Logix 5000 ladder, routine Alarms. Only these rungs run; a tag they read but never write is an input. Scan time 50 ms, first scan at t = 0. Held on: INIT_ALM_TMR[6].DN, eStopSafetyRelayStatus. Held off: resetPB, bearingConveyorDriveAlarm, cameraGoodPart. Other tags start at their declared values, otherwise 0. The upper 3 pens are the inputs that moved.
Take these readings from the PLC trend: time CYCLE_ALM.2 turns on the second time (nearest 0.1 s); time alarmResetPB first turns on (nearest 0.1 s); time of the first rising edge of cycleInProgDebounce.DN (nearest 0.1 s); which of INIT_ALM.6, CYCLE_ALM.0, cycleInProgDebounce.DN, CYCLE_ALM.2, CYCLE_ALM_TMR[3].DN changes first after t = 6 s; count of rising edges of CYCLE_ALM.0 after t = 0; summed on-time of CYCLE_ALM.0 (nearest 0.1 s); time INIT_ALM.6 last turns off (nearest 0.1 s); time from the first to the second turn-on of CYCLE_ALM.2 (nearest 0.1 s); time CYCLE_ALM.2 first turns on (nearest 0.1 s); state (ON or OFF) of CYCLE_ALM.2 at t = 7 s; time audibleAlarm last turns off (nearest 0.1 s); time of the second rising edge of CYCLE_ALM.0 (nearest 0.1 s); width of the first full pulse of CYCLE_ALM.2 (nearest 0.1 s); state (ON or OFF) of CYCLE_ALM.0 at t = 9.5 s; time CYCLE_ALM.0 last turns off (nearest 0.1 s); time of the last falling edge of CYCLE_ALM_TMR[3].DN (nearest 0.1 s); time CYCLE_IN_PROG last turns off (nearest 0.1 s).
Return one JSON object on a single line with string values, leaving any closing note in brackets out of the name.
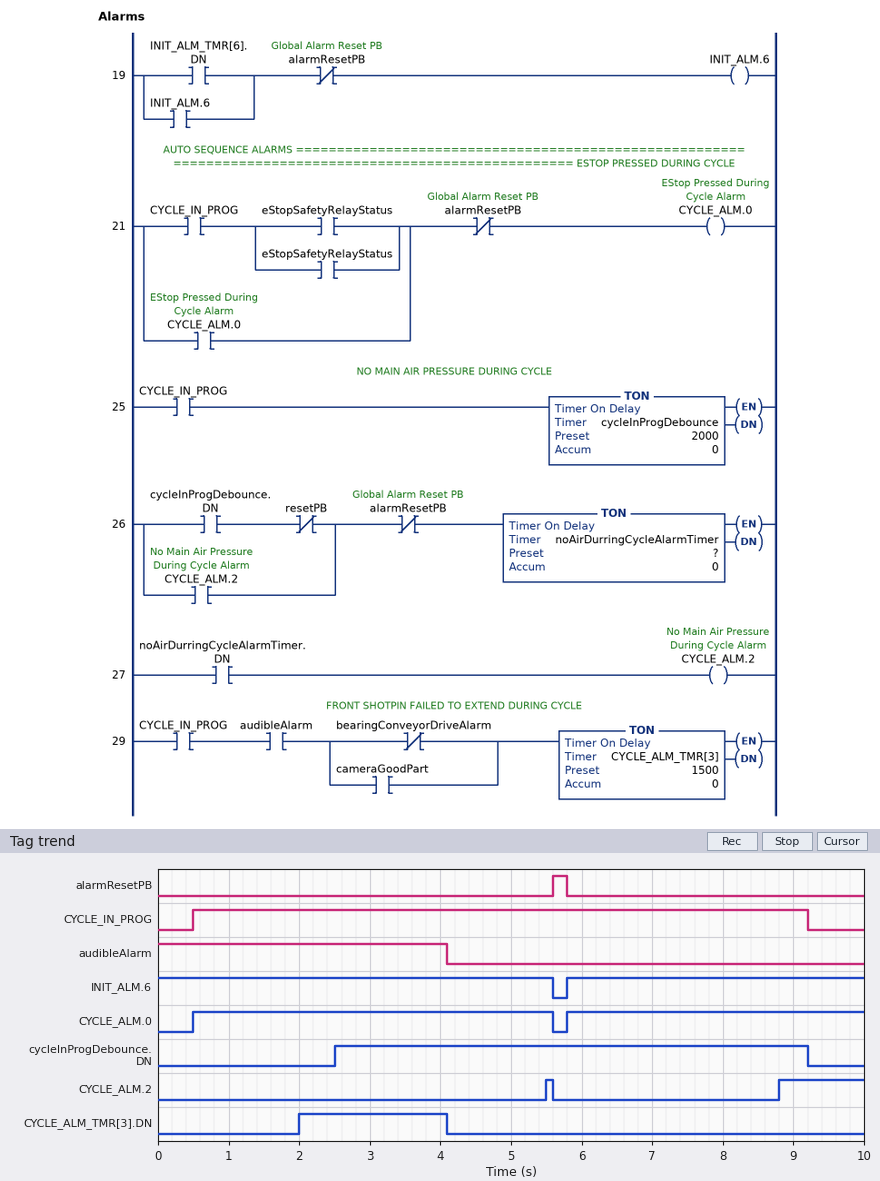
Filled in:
{"time CYCLE_ALM.2 turns on the second time": "8.8 s", "time alarmResetPB first turns on": "5.6 s", "time of the first rising edge of cycleInProgDebounce.DN": "2.5 s", "which of INIT_ALM.6, CYCLE_ALM.0, cycleInProgDebounce.DN, CYCLE_ALM.2, CYCLE_ALM_TMR[3].DN changes first after t = 6 s": "CYCLE_ALM.2", "count of rising edges of CYCLE_ALM.0 after t = 0": "2", "summed on-time of CYCLE_ALM.0": "9.3 s", "time INIT_ALM.6 last turns off": "5.6 s", "time from the first to the second turn-on of CYCLE_ALM.2": "3.3 s", "time CYCLE_ALM.2 first turns on": "5.5 s", "state (ON or OFF) of CYCLE_ALM.2 at t = 7 s": "OFF", "time audibleAlarm last turns off": "4.1 s", "time of the second rising edge of CYCLE_ALM.0": "5.8 s", "width of the first full pulse of CYCLE_ALM.2": "0.1 s", "state (ON or OFF) of CYCLE_ALM.0 at t = 9.5 s": "ON", "time CYCLE_ALM.0 last turns off": "5.6 s", "time of the last falling edge of CYCLE_ALM_TMR[3].DN": "4.1 s", "time CYCLE_IN_PROG last turns off": "9.2 s"}
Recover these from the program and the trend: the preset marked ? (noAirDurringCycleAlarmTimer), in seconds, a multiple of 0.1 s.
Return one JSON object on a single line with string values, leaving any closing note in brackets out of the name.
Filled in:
{"the preset marked ? (noAirDurringCycleAlarmTimer), in seconds, a multiple of 0.1 s": "3.0 s"}
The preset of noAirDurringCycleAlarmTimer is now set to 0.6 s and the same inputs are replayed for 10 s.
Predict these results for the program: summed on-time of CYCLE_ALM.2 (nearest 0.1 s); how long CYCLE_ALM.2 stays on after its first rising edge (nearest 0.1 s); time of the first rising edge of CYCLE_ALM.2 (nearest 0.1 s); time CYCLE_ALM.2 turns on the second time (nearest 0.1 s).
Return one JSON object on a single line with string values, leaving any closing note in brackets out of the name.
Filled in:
{"summed on-time of CYCLE_ALM.2": "6.1 s", "how long CYCLE_ALM.2 stays on after its first rising edge": "2.5 s", "time of the first rising edge of CYCLE_ALM.2": "3.1 s", "time CYCLE_ALM.2 turns on the second time": "6.4 s"}
